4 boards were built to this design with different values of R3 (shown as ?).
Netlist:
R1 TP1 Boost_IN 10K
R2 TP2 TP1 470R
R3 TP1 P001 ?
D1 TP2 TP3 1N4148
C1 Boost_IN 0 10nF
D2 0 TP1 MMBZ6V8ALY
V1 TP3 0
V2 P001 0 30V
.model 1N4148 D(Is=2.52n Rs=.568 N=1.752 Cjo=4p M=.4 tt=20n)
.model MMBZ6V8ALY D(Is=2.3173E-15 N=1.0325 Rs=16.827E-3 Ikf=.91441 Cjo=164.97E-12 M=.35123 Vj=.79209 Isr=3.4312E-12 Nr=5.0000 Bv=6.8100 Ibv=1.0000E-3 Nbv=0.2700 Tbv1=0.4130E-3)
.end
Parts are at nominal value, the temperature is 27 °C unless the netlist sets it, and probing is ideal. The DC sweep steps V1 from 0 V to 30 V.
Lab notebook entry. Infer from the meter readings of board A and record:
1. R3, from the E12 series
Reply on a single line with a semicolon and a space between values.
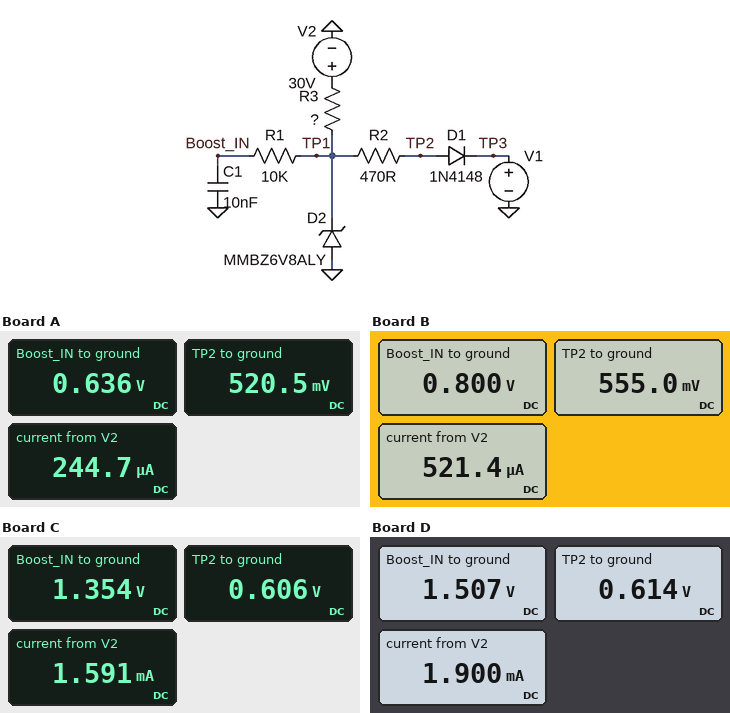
120 kΩ
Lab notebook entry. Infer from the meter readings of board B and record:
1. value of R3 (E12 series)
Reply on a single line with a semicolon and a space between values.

56 kΩ
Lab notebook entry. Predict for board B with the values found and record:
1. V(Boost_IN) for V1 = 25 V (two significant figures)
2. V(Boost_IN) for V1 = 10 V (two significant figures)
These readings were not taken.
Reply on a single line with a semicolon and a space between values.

6.8 V; 6.8 V
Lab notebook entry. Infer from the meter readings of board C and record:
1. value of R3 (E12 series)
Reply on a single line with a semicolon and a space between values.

18 kΩ
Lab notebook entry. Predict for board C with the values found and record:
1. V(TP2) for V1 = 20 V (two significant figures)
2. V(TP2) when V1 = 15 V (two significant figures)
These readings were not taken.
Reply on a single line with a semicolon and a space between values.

6.8 V; 6.8 V
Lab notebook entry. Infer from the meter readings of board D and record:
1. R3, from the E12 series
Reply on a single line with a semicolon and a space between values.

15 kΩ
